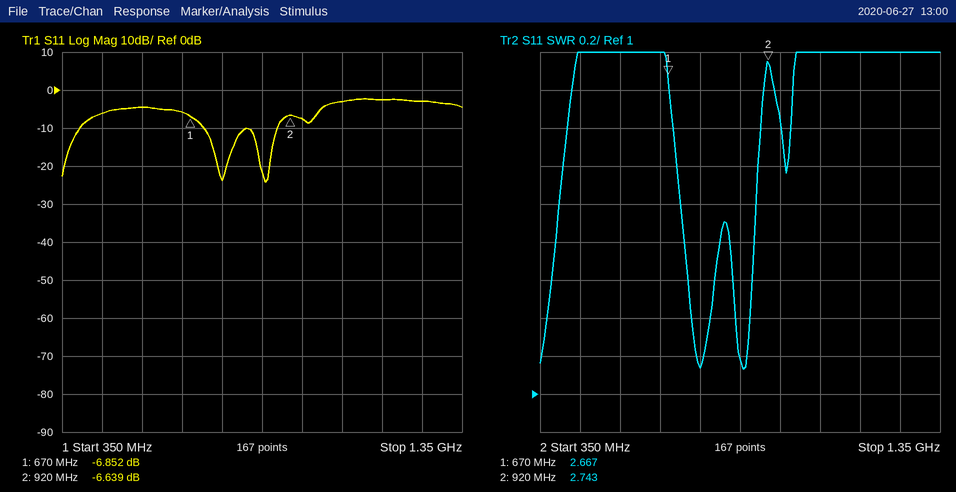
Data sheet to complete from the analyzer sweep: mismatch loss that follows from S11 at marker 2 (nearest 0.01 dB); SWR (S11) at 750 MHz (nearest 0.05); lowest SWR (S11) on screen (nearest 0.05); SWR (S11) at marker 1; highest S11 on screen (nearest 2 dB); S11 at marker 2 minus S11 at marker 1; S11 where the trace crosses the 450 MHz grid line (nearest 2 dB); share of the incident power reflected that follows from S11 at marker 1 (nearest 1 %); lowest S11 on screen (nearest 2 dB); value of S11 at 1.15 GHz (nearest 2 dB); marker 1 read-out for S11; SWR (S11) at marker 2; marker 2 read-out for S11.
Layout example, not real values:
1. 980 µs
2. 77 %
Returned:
1. 1.06 dB
2. 1.15
3. 1.15
4. 2.667
5. -2 dB
6. 0.213 dB
7. -6 dB
8. 21 %
9. -24 dB
10. -2 dB
11. -6.852 dB
12. 2.743
13. -6.639 dB
